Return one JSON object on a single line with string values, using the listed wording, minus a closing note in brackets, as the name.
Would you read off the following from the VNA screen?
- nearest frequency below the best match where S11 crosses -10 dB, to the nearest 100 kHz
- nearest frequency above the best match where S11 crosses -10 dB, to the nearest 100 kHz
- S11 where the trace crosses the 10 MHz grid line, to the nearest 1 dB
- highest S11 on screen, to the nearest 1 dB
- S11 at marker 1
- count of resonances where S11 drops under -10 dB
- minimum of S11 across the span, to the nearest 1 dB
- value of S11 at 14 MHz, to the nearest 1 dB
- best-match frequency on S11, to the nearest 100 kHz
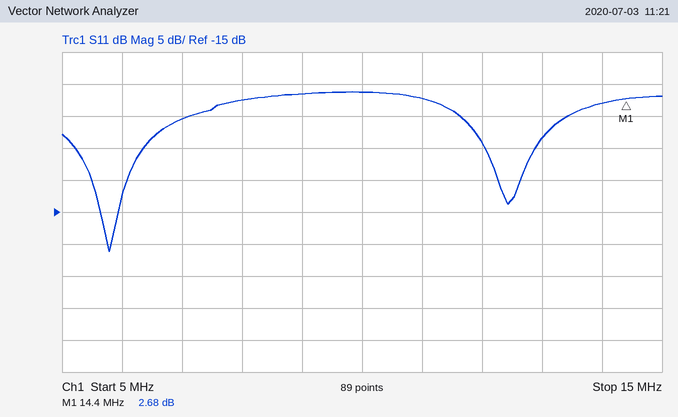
{"nearest frequency below the best match where S11 crosses -10 dB, to the nearest 100 kHz": "5.5 MHz", "nearest frequency above the best match where S11 crosses -10 dB, to the nearest 100 kHz": "6.1 MHz", "S11 where the trace crosses the 10 MHz grid line, to the nearest 1 dB": "4 dB", "highest S11 on screen, to the nearest 1 dB": "4 dB", "S11 at marker 1": "2.68 dB", "count of resonances where S11 drops under -10 dB": "2", "minimum of S11 across the span, to the nearest 1 dB": "-21 dB", "value of S11 at 14 MHz, to the nearest 1 dB": "2 dB", "best-match frequency on S11, to the nearest 100 kHz": "5.8 MHz"}
